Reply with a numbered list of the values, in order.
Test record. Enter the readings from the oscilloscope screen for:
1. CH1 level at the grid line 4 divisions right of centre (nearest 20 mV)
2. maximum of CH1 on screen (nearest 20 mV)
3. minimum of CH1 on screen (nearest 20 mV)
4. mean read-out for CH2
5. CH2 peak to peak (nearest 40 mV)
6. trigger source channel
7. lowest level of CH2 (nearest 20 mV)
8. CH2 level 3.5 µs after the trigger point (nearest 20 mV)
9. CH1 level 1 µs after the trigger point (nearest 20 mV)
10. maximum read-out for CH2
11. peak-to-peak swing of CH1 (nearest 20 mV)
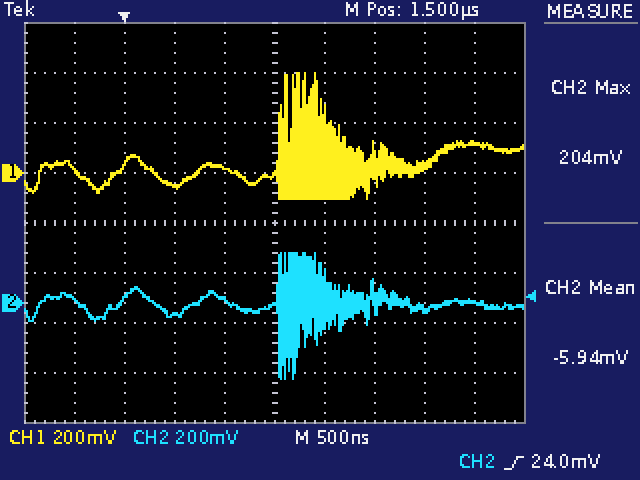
1. 120 mV
2. 400 mV
3. -100 mV
4. -5.94 mV
5. 520 mV
6. CH2
7. -300 mV
8. 0 mV
9. 20 mV
10. 204 mV
11. 500 mV
